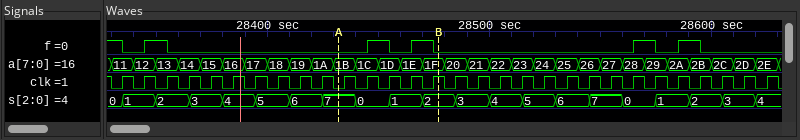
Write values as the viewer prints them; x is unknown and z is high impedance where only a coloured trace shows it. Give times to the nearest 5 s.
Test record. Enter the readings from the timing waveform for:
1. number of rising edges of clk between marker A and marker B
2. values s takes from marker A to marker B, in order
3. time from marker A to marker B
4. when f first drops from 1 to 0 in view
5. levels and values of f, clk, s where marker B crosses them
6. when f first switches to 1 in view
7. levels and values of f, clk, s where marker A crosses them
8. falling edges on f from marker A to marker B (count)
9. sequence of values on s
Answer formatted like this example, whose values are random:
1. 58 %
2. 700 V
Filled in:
1. 5
2. 7, 0, 1, 2
3. 45 s
4. 28335 s
5. f=0, clk=1, s=2
6. 28345 s
7. f=0, clk=0, s=7
8. 2
9. 0, 1, 2, 3, 4, 5, 6, 7, 0, 1, 2, 3, 4, 5, 6, 7, 0, 1, 2, 3, 4
